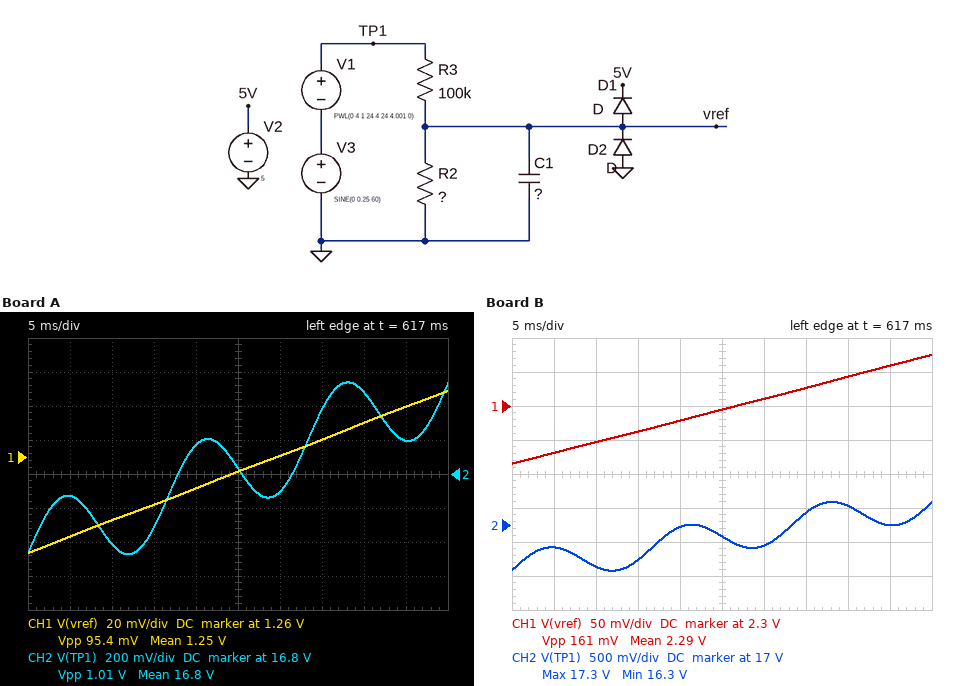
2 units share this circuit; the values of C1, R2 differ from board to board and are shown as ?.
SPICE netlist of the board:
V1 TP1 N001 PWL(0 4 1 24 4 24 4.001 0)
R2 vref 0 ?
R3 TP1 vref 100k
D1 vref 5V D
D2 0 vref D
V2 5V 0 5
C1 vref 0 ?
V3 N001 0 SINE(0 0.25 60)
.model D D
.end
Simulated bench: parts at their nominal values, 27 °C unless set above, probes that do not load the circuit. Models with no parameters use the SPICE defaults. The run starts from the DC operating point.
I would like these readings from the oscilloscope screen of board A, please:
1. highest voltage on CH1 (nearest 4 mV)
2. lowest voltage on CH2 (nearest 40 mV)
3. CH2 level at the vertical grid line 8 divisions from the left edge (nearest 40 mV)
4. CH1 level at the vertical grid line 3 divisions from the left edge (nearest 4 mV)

1.300 V
16.32 V
17.28 V
1.232 V
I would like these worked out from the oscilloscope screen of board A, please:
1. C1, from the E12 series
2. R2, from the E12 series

27 µF
12 kΩ
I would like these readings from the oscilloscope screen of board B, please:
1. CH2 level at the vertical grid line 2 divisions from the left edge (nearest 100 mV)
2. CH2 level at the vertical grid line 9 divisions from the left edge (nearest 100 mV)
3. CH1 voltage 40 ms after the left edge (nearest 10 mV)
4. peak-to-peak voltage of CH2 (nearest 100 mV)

16.4 V
17.0 V
2.34 V
1.0 V
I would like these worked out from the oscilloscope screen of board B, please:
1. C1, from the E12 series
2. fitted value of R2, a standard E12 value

27 µF
39 kΩ
